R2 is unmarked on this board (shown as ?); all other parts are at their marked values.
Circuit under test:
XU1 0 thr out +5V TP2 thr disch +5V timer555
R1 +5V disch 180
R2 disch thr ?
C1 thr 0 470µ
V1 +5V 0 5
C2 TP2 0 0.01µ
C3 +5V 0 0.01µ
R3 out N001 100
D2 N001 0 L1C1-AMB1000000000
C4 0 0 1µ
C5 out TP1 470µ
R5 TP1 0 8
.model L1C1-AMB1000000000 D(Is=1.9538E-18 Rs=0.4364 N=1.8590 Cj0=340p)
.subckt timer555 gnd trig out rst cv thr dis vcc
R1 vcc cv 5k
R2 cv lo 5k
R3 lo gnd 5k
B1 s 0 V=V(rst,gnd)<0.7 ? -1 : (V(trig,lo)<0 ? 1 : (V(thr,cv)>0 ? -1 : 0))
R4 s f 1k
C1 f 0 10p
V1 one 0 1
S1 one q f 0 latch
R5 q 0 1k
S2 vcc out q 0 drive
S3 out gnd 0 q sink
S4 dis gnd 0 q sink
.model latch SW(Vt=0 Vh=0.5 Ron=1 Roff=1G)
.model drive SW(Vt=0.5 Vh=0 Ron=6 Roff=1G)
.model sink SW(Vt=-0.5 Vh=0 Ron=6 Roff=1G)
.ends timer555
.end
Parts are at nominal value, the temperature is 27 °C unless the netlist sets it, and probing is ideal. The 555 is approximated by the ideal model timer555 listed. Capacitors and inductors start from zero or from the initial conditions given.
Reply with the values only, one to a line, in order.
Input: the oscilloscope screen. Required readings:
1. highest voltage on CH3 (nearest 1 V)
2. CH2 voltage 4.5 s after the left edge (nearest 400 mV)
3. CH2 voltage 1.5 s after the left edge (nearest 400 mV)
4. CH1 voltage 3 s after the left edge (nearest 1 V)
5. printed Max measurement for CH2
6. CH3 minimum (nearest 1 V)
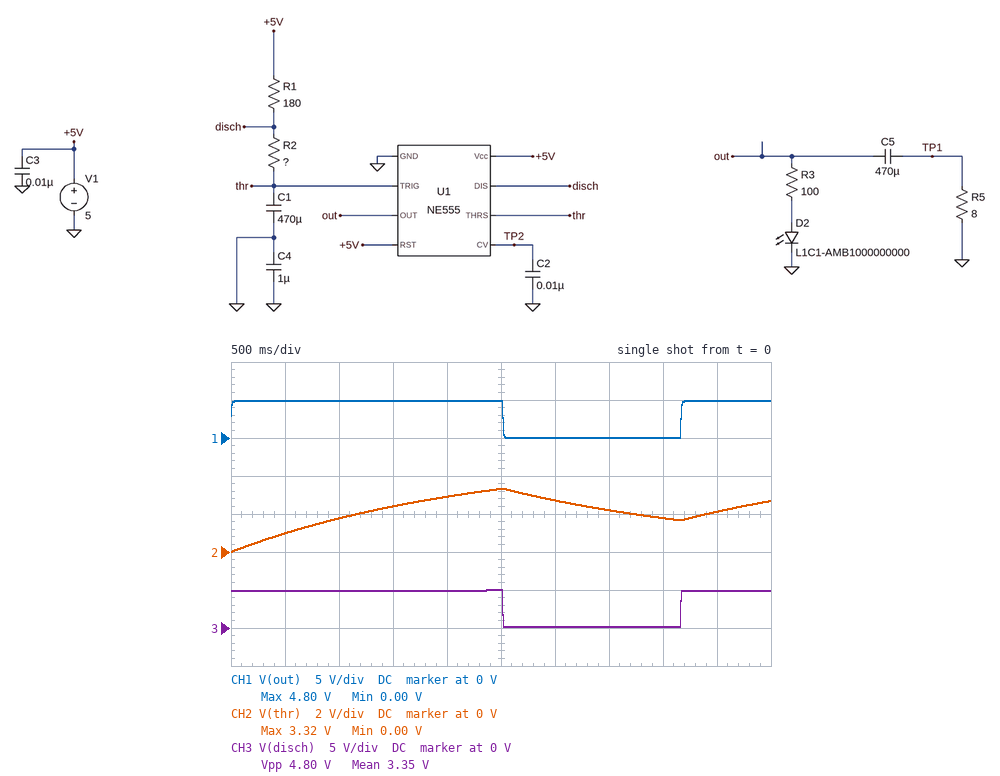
5 V
2.0 V
2.4 V
0 V
3.32 V
0 V
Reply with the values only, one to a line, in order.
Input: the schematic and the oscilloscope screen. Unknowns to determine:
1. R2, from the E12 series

4.7 kΩ
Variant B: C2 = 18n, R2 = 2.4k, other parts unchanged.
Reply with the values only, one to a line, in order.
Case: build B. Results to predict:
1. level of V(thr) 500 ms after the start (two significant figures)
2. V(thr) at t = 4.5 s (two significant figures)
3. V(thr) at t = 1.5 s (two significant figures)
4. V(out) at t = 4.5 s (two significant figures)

1.7 V
3.0 V
2.9 V
4.8 V
